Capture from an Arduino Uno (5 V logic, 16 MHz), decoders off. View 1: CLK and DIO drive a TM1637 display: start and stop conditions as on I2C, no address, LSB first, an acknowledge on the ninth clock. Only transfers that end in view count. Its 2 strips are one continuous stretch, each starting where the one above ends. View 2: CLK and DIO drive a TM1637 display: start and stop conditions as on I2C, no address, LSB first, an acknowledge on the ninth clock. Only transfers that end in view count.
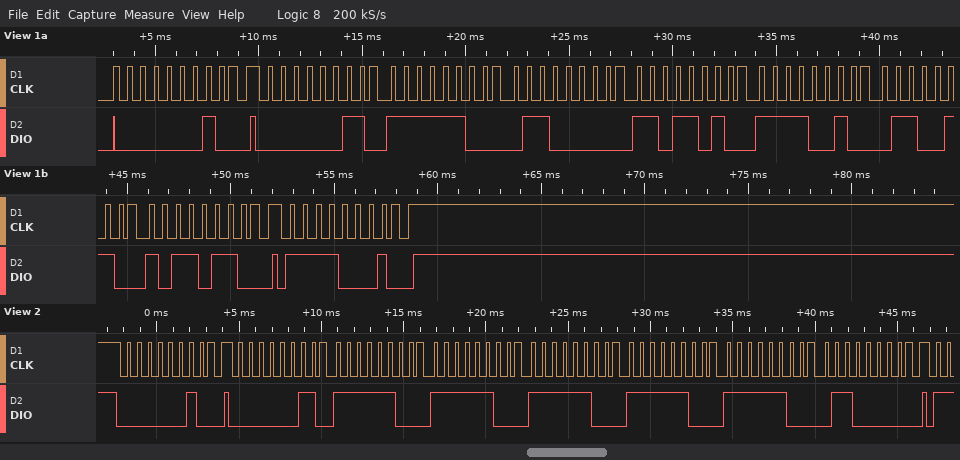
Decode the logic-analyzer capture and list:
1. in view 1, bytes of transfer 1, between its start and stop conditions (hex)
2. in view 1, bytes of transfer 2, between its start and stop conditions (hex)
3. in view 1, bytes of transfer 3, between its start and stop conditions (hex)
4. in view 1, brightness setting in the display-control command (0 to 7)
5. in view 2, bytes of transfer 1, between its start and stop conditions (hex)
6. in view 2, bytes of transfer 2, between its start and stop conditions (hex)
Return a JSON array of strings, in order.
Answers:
["40", "C0 3F 06 5B 4F 66 6D", "8F", "7", "40", "C0 3F 3F 3F 3F 3F 06"]
